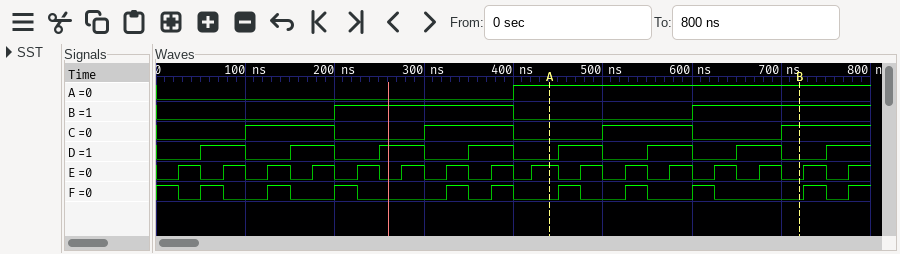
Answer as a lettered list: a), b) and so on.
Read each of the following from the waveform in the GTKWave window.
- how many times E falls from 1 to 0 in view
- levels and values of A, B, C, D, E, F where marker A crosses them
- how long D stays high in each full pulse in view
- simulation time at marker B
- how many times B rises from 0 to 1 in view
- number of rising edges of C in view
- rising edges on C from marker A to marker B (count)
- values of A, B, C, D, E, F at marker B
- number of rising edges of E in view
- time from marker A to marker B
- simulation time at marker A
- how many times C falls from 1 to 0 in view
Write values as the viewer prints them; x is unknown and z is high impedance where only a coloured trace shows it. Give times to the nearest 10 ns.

a) 15
b) A=1, B=0, C=0, D=0, E=1, F=0
c) 50 ns, 50 ns, 50 ns, 50 ns, 50 ns, 50 ns, 50 ns
d) 720 ns
e) 2
f) 4
g) 2
h) A=1, B=1, C=1, D=0, E=0, F=0
i) 16
j) 280 ns
k) 440 ns
l) 3
